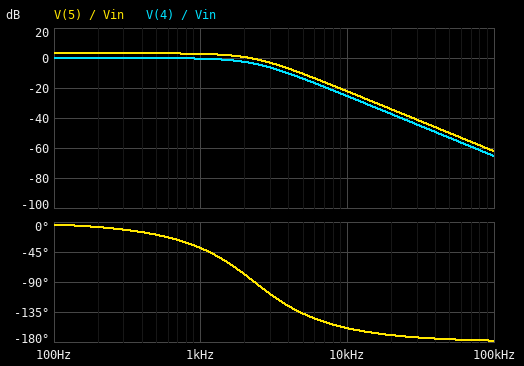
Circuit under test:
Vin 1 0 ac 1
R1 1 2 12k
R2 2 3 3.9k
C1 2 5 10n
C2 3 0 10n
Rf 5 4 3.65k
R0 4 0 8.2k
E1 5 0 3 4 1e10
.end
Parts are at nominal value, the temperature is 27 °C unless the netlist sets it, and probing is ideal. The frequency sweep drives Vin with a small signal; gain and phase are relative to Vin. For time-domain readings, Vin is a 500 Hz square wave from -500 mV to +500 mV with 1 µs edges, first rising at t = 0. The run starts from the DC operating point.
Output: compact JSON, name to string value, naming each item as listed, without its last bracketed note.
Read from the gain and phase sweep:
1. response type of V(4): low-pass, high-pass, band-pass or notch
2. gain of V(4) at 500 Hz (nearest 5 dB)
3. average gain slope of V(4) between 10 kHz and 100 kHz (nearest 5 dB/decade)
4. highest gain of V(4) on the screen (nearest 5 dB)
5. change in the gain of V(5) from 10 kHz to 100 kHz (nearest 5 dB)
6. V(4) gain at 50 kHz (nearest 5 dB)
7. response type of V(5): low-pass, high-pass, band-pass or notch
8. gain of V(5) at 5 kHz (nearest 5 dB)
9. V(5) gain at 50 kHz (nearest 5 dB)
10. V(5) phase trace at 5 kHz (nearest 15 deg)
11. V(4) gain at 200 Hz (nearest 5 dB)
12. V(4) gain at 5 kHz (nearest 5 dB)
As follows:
{"response type of V(4): low-pass, high-pass, band-pass or notch": "low-pass", "gain of V(4) at 500 Hz": "0 dB", "average gain slope of V(4) between 10 kHz and 100 kHz": "-40 dB/decade", "highest gain of V(4) on the screen": "0 dB", "change in the gain of V(5) from 10 kHz to 100 kHz": "-40 dB", "V(4) gain at 50 kHz": "-55 dB", "response type of V(5): low-pass, high-pass, band-pass or notch": "low-pass", "gain of V(5) at 5 kHz": "-10 dB", "V(5) gain at 50 kHz": "-50 dB", "V(5) phase trace at 5 kHz": "-135 deg", "V(4) gain at 200 Hz": "0 dB", "V(4) gain at 5 kHz": "-15 dB"}
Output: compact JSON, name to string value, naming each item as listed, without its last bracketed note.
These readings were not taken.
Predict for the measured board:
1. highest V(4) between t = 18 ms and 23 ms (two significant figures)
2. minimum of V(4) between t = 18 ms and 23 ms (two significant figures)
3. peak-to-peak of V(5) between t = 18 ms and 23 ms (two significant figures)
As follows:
{"highest V(4) between t = 18 ms and 23 ms": "520 mV", "minimum of V(4) between t = 18 ms and 23 ms": "-520 mV", "peak-to-peak of V(5) between t = 18 ms and 23 ms": "1.5 V"}
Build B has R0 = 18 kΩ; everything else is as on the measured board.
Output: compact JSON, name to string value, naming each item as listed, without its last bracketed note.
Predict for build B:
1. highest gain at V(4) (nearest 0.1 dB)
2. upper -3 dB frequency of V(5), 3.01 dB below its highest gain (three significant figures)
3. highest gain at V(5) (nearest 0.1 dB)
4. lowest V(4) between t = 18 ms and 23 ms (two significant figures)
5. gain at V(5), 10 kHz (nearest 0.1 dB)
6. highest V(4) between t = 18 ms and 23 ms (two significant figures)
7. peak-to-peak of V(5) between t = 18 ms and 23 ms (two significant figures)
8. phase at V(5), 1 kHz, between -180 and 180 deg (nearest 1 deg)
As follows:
{"highest gain at V(4)": "0 dB", "upper -3 dB frequency of V(5), 3.01 dB below its highest gain": "1.53 kHz", "highest gain at V(5)": "1.6 dB", "lowest V(4) between t = 18 ms and 23 ms": "-500 mV", "gain at V(5), 10 kHz": "-24.2 dB", "highest V(4) between t = 18 ms and 23 ms": "500 mV", "peak-to-peak of V(5) between t = 18 ms and 23 ms": "1.2 V", "phase at V(5), 1 kHz, between -180 and 180 deg": "-46 deg"}
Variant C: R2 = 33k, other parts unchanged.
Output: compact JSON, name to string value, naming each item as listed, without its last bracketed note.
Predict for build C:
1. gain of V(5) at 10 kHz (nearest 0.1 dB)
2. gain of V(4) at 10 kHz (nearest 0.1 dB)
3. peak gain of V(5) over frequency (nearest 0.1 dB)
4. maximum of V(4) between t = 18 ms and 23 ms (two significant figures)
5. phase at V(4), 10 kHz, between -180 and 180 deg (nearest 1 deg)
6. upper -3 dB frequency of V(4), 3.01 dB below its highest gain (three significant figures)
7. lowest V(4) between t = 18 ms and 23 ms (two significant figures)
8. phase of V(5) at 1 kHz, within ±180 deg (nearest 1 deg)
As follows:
{"gain of V(5) at 10 kHz": "-40.7 dB", "gain of V(4) at 10 kHz": "-43.9 dB", "peak gain of V(5) over frequency": "3.2 dB", "maximum of V(4) between t = 18 ms and 23 ms": "460 mV", "phase at V(4), 10 kHz, between -180 and 180 deg": "-171 deg", "upper -3 dB frequency of V(4), 3.01 dB below its highest gain": "517 Hz", "lowest V(4) between t = 18 ms and 23 ms": "-460 mV", "phase of V(5) at 1 kHz, within ±180 deg": "-103 deg"}
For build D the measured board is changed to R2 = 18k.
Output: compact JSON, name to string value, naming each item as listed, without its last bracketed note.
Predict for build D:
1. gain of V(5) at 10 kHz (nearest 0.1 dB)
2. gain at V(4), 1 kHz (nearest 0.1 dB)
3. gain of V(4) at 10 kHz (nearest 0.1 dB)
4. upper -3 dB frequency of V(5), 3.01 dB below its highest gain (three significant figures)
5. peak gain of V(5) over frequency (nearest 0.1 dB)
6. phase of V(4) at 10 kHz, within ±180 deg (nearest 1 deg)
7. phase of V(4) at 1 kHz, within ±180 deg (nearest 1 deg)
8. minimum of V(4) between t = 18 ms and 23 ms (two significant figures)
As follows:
{"gain of V(5) at 10 kHz": "-35.5 dB", "gain at V(4), 1 kHz": "-3.8 dB", "gain of V(4) at 10 kHz": "-38.7 dB", "upper -3 dB frequency of V(5), 3.01 dB below its highest gain": "888 Hz", "peak gain of V(5) over frequency": "3.2 dB", "phase of V(4) at 10 kHz, within ±180 deg": "-170 deg", "phase of V(4) at 1 kHz, within ±180 deg": "-85 deg", "minimum of V(4) between t = 18 ms and 23 ms": "-510 mV"}
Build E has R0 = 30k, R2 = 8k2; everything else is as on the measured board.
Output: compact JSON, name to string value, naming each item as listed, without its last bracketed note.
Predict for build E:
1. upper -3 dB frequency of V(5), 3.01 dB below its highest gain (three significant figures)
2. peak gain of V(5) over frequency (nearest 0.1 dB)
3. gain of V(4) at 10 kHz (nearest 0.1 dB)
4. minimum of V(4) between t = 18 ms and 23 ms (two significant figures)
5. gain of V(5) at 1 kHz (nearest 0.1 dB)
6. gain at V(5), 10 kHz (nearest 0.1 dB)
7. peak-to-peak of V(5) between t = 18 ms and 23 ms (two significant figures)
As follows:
{"upper -3 dB frequency of V(5), 3.01 dB below its highest gain": "1.12 kHz", "peak gain of V(5) over frequency": "1.0 dB", "gain of V(4) at 10 kHz": "-32.0 dB", "minimum of V(4) between t = 18 ms and 23 ms": "-500 mV", "gain of V(5) at 1 kHz": "-1.5 dB", "gain at V(5), 10 kHz": "-31.0 dB", "peak-to-peak of V(5) between t = 18 ms and 23 ms": "1.1 V"}
